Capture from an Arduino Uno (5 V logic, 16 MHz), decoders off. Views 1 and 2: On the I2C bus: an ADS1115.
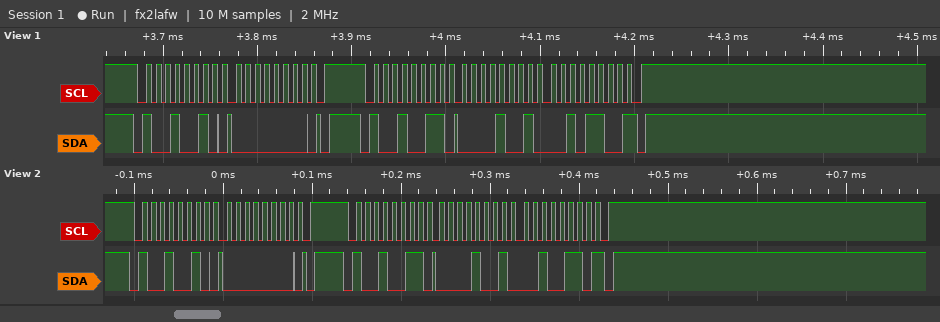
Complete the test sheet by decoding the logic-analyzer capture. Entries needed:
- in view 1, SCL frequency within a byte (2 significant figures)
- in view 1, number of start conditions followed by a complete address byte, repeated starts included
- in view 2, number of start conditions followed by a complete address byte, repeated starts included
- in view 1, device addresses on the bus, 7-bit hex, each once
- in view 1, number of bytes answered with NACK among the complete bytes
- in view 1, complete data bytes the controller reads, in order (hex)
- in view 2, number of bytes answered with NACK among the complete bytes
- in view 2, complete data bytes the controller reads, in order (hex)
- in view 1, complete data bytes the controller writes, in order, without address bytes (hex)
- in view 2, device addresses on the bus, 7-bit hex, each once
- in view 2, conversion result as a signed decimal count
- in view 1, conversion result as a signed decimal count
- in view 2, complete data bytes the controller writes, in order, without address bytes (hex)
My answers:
100 kHz
2
2
0x49
1
09 2C
1
09 26
00
0x49
2342
2348
00
